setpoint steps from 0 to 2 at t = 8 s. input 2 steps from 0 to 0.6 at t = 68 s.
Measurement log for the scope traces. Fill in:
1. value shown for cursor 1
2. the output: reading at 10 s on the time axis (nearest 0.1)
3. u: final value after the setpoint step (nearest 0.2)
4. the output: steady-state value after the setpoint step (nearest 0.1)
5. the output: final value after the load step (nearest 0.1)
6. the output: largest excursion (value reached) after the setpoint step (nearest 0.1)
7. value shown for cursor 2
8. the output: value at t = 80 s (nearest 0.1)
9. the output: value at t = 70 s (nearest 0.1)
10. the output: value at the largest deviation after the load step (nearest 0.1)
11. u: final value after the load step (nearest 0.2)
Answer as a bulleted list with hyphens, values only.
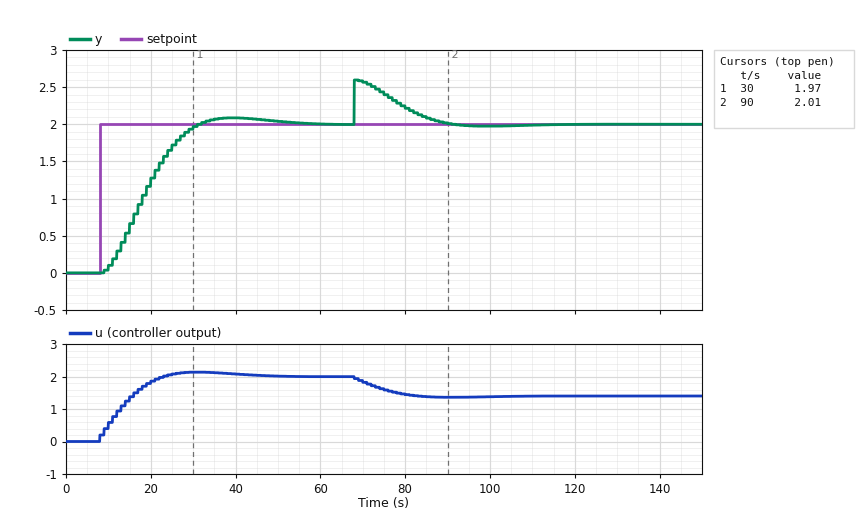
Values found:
- 1.97
- 0.1
- 2.0
- 2.0
- 2.0
- 2.1
- 2.01
- 2.2
- 2.6
- 2.6
- 1.4
